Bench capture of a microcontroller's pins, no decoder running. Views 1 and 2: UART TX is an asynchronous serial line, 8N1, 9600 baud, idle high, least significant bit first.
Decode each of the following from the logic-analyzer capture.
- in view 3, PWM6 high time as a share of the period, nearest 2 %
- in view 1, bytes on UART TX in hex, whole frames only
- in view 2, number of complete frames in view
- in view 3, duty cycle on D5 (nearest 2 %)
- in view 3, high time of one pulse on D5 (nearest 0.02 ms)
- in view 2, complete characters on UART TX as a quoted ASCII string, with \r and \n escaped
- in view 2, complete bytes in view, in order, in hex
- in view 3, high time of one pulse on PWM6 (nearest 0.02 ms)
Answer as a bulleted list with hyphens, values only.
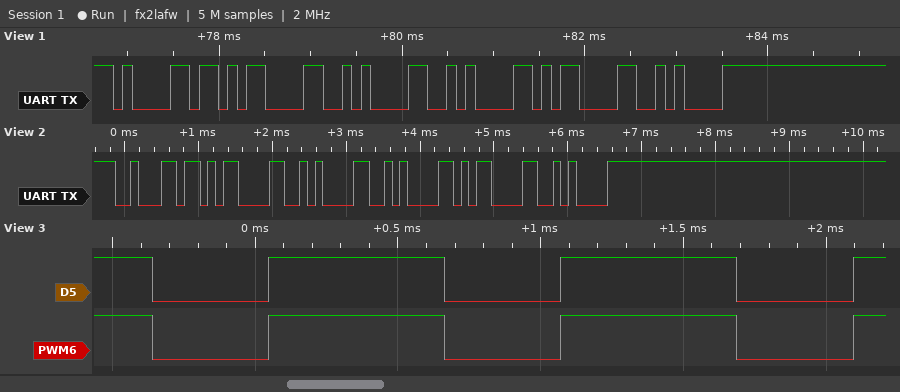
- 60 %
- 0x61 0x0D 0x0A 0x0A 0x0D 0x0A
- 6
- 60 %
- 0.62 ms
- "b\r\n\n\r\n"
- 62 0D 0A 0A 0D 0A
- 0.62 ms
